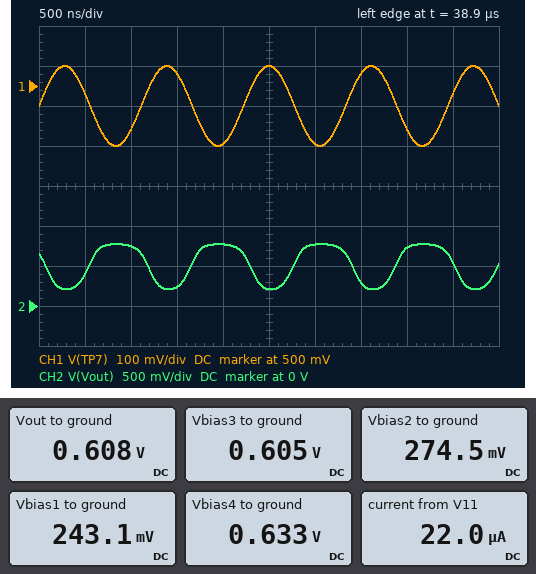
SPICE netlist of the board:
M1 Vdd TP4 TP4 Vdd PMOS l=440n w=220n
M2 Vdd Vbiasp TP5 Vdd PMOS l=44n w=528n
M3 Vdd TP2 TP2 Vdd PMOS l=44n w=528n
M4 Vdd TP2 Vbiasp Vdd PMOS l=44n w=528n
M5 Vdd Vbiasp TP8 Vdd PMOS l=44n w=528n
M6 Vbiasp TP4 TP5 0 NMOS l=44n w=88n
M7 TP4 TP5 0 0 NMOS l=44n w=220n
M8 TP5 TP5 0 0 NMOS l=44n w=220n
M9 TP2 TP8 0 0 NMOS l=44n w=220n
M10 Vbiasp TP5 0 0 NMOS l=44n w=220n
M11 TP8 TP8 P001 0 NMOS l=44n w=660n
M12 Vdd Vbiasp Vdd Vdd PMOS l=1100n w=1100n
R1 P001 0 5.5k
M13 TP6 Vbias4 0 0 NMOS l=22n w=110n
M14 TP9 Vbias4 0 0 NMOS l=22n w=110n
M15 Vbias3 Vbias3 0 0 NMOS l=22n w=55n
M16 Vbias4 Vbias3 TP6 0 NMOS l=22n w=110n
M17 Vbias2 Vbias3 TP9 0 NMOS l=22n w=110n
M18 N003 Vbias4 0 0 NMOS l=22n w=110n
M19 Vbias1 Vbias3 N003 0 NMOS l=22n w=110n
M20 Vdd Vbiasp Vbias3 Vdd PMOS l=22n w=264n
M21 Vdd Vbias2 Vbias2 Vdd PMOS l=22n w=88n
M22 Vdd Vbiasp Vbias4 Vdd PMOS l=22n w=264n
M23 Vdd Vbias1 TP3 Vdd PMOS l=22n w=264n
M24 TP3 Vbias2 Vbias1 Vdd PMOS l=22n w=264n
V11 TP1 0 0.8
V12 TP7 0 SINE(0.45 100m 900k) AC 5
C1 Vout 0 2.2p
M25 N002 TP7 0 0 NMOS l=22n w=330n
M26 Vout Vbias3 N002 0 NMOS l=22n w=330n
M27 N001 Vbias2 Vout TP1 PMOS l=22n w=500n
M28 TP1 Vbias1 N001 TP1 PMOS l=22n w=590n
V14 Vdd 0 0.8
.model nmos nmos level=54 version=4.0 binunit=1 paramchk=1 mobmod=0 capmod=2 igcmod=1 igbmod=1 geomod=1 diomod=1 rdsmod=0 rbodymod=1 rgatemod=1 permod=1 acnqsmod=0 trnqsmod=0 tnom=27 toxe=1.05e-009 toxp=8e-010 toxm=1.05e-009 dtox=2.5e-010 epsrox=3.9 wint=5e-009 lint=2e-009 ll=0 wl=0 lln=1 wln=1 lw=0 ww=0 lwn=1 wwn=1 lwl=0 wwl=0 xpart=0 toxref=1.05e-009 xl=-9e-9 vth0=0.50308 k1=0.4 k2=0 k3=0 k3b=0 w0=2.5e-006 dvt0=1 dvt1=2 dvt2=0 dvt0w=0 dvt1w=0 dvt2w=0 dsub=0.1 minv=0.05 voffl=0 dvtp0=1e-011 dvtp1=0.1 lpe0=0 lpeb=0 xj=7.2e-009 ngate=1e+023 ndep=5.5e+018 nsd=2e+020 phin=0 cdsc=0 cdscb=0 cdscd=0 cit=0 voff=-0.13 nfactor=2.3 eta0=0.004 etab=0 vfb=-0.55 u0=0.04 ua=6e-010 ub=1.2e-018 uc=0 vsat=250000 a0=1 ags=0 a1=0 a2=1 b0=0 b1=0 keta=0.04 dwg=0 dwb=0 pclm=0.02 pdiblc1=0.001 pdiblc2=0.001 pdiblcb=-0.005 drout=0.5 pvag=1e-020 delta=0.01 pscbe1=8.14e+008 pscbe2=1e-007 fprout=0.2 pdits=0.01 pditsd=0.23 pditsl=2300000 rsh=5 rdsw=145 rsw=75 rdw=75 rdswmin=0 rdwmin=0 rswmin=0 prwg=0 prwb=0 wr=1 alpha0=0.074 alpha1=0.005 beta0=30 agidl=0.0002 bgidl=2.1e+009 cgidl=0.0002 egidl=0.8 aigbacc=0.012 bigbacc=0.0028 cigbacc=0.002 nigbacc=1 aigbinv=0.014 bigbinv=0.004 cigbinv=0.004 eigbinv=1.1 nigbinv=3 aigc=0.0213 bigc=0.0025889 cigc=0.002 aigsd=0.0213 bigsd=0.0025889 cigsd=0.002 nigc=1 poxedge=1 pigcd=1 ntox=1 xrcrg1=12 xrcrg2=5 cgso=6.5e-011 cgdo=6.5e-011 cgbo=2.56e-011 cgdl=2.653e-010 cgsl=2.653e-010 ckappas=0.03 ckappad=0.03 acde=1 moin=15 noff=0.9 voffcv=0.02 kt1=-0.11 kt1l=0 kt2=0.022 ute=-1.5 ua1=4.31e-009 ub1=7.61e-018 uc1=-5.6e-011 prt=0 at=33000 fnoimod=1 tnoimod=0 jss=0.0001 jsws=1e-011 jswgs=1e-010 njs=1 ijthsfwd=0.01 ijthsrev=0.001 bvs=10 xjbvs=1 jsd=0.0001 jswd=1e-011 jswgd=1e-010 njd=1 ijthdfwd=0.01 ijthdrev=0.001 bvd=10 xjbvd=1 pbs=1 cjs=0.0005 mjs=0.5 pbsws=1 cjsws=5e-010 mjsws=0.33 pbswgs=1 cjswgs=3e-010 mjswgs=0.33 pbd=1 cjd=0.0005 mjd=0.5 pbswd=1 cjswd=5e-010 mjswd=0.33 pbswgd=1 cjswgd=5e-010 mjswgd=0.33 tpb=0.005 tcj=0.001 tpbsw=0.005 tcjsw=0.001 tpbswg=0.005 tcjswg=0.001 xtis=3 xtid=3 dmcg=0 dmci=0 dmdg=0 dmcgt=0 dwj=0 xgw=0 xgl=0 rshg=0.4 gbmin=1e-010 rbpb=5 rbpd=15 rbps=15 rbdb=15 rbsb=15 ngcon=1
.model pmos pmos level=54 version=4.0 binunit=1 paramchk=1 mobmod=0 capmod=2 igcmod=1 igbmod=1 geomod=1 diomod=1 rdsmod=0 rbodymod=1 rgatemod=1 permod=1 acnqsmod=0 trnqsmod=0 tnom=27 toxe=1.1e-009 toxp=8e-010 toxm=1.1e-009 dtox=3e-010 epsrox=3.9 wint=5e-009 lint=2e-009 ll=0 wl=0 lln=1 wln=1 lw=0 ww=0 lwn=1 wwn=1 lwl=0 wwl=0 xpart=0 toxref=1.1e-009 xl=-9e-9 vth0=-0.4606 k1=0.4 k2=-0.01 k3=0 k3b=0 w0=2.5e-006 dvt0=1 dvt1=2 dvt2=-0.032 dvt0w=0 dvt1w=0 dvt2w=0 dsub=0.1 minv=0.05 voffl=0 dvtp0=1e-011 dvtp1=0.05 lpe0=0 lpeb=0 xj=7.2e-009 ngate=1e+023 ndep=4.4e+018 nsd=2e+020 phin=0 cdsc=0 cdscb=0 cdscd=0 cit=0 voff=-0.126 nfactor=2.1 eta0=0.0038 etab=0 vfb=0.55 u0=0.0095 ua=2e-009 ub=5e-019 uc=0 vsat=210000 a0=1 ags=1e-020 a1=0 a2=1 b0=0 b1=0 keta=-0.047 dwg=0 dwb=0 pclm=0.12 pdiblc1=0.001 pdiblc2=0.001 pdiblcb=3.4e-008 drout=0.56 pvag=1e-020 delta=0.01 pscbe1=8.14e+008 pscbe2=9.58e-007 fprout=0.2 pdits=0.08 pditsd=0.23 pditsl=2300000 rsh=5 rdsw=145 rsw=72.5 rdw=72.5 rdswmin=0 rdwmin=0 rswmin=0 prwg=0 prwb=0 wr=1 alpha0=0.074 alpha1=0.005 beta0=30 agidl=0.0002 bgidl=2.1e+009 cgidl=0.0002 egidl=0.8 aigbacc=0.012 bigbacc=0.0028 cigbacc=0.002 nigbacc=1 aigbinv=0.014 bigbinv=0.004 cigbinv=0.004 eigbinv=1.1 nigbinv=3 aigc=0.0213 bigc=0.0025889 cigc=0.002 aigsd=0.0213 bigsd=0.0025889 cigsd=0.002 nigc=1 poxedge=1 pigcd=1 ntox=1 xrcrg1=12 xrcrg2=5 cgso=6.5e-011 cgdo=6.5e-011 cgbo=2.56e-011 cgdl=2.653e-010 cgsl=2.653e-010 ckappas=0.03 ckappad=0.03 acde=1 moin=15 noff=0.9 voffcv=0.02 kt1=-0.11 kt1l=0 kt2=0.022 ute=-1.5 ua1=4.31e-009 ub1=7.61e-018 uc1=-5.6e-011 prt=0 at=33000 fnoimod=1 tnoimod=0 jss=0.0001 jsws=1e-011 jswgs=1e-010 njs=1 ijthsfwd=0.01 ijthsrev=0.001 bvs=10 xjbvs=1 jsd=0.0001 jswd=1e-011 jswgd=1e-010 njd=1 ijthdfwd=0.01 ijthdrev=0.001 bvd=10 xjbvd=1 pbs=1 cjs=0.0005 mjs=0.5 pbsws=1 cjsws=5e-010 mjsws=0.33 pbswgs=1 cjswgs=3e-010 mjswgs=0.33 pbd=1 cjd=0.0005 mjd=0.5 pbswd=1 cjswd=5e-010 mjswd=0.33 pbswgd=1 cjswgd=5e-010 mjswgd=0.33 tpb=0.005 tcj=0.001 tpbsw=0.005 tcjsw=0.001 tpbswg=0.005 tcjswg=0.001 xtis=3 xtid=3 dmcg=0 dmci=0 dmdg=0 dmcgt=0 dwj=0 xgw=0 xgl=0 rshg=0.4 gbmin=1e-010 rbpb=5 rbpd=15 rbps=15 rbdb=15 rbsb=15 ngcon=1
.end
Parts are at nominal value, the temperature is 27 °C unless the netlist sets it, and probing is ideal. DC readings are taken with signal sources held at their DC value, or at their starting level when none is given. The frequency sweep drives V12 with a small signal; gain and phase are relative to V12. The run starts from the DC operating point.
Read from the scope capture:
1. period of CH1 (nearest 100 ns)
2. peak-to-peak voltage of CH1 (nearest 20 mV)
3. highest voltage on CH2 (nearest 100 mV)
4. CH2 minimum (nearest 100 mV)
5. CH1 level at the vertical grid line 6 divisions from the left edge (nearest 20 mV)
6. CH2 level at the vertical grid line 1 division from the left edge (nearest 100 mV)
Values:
1.1 µs
200 mV
800 mV
200 mV
360 mV
400 mV
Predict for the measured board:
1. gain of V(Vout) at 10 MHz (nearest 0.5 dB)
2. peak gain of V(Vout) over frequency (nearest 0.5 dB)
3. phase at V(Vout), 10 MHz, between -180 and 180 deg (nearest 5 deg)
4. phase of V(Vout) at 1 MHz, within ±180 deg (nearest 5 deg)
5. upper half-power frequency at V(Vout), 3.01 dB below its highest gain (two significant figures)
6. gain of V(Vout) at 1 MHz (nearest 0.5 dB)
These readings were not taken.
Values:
5.5 dB
12.0 dB
115 deg
170 deg
5.1 MHz
12.0 dB
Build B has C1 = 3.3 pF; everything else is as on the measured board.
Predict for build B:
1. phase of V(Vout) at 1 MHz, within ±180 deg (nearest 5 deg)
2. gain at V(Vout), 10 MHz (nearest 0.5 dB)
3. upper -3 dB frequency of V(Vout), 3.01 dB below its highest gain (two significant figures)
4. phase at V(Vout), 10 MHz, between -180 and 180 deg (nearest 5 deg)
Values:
165 deg
2.5 dB
3.4 MHz
110 deg
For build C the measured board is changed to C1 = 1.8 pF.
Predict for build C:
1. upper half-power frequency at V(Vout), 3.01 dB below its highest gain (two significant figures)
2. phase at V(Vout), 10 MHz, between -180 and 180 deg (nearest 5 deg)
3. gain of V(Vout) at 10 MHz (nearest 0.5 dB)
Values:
6.3 MHz
120 deg
6.5 dB
